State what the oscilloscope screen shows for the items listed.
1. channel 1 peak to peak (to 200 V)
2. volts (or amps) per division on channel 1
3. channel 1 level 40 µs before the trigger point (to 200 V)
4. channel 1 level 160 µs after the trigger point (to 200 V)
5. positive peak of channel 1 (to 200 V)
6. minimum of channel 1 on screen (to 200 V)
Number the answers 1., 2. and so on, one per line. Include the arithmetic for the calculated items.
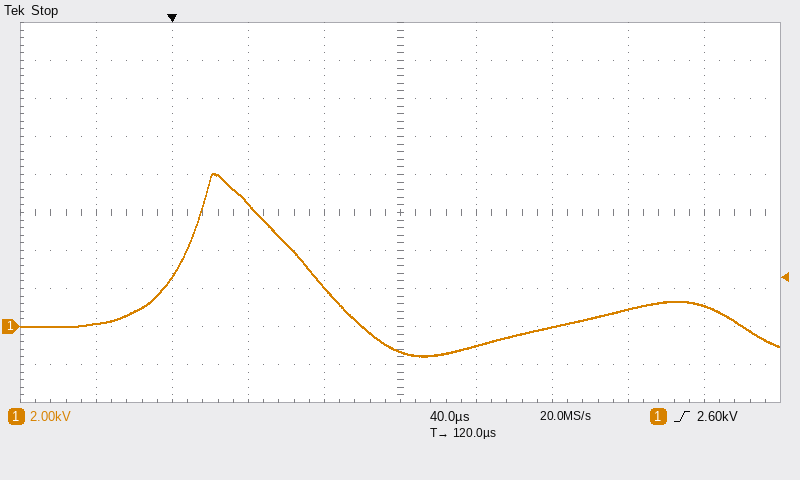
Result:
1. 8.0 kV − (-1.6 kV) = 9.6 kV
2. 2 kV
3. 200 V
4. -1.0 kV
5. 8.0 kV
6. -1.6 kV
